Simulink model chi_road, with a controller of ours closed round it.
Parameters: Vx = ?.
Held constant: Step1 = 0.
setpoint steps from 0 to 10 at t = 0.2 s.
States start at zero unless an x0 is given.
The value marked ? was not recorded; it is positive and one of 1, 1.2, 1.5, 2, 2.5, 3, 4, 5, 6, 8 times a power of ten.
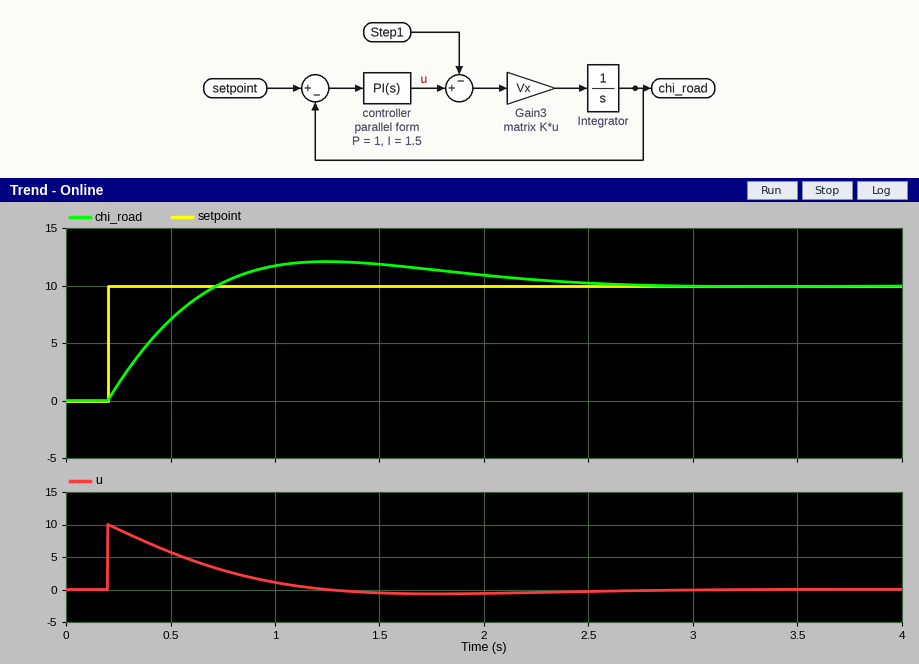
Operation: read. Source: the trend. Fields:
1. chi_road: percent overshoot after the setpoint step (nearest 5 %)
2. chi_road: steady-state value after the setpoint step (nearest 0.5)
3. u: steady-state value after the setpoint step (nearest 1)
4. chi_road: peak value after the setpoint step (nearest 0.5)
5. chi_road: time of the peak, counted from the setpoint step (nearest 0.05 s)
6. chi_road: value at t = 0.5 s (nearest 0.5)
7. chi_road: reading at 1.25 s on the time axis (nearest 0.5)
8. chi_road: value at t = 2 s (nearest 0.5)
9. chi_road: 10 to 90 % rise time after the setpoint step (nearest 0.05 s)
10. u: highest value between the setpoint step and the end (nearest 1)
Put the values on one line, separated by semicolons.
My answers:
20 %; 10.0; 0; 12.0; 1.05 s; 7.0; 12.0; 11.0; 0.40 s; 10
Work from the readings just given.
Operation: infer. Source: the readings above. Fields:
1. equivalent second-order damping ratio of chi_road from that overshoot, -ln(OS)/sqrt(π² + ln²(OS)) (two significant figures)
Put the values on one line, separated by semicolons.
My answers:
0.46
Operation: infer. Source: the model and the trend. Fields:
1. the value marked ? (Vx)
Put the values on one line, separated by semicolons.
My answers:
3
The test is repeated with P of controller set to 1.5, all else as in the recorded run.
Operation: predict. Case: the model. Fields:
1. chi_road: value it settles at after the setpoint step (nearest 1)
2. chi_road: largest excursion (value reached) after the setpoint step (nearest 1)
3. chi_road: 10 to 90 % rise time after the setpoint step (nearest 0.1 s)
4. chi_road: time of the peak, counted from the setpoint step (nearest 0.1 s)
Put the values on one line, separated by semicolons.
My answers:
10; 11; 0.3 s; 0.9 s
